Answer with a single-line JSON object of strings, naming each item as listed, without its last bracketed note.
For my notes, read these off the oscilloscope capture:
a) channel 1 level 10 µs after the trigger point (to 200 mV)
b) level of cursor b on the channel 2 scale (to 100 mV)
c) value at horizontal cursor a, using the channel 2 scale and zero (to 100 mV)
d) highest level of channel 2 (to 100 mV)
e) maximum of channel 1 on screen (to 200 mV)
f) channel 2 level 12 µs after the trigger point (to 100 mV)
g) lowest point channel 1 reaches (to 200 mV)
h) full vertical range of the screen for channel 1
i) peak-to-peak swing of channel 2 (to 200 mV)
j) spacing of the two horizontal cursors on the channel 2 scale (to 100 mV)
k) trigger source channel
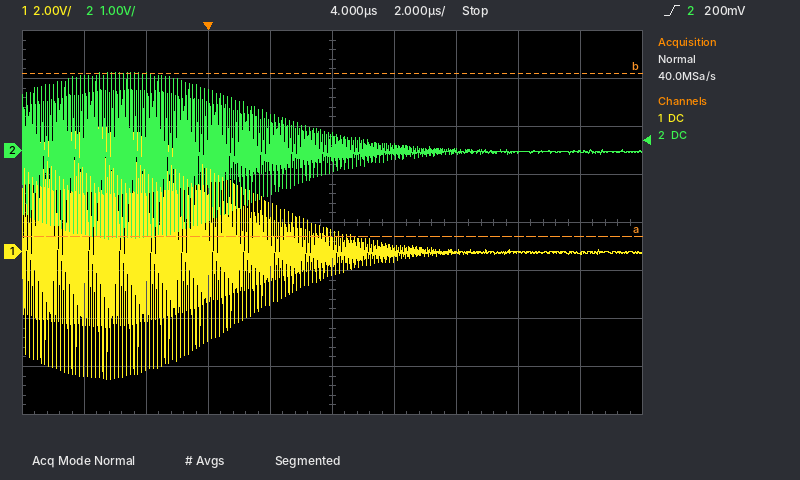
{"channel 1 level 10 µs after the trigger point": "0.0 V", "level of cursor b on the channel 2 scale": "1.6 V", "value at horizontal cursor a, using the channel 2 scale and zero": "-1.8 V", "highest level of channel 2": "1.6 V", "maximum of channel 1 on screen": "5.2 V", "channel 2 level 12 µs after the trigger point": "0.0 V", "lowest point channel 1 reaches": "-5.4 V", "full vertical range of the screen for channel 1": "16 V", "peak-to-peak swing of channel 2": "3.4 V", "spacing of the two horizontal cursors on the channel 2 scale": "3.4 V", "trigger source channel": "channel 2"}
